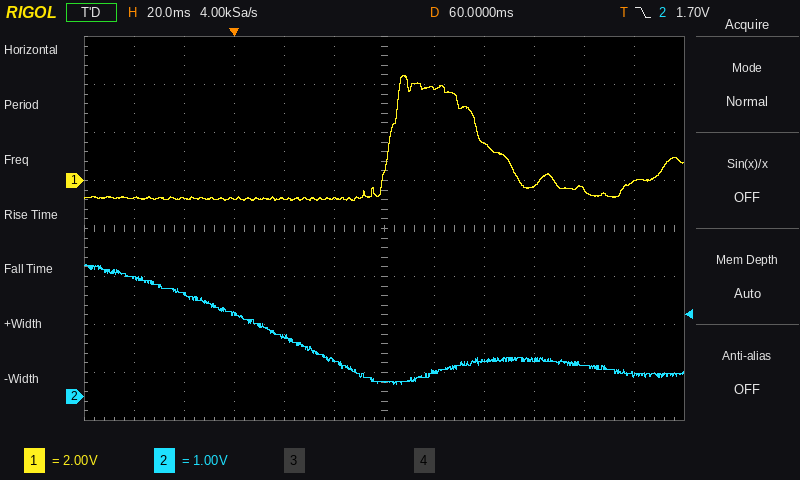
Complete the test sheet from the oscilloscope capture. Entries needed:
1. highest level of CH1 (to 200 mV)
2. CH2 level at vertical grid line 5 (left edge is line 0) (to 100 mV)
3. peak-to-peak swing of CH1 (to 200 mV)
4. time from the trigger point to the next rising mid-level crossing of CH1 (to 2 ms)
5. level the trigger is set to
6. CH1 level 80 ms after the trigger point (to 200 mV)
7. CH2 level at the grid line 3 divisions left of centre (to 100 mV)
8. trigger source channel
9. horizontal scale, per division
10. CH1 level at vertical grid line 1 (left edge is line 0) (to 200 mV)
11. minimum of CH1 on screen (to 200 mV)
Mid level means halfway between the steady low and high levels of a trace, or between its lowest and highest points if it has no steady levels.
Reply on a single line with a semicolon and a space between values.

4.4 V; 800 mV; 5.2 V; 62 ms; 1.70 V; 3.8 V; 1.7 V; CH2; 20 ms; -800 mV; -800 mV
